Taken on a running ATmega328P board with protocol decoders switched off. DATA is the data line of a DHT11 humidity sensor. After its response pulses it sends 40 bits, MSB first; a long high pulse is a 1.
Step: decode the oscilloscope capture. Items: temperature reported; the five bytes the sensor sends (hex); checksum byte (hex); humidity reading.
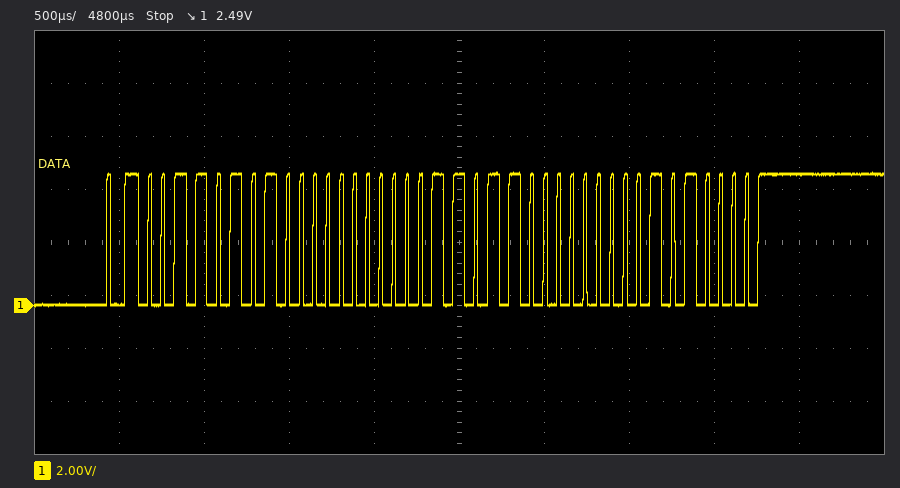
27.0 °C
35 00 1B 00 50
0x50
53 %
